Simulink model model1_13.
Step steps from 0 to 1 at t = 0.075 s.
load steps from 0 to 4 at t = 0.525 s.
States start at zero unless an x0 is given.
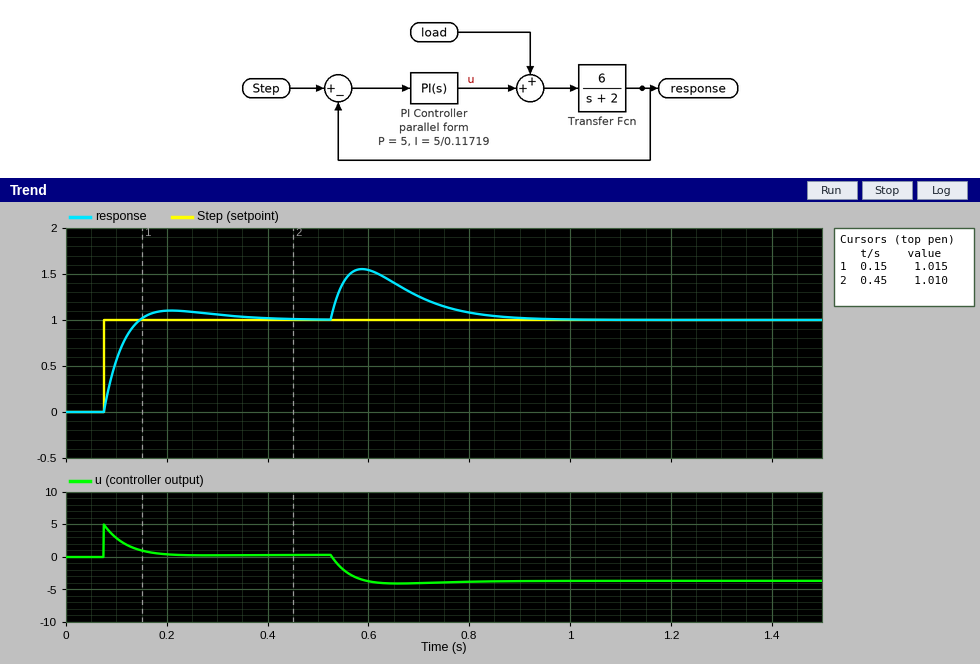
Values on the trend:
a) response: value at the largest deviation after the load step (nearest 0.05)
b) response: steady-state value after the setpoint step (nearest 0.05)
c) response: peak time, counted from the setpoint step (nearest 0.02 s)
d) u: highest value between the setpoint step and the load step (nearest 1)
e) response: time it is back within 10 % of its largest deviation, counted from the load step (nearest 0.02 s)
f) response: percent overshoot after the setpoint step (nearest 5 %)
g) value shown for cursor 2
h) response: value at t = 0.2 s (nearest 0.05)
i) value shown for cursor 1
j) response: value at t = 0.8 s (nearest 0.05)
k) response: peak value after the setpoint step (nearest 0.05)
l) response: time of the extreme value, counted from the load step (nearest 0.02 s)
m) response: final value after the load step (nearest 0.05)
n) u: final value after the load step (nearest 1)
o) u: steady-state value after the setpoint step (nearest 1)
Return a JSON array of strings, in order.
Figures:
["1.55", "1.00", "0.14 s", "5", "0.30 s", "10 %", "1.010", "1.10", "1.015", "1.10", "1.10", "0.06 s", "1.00", "-4", "0"]
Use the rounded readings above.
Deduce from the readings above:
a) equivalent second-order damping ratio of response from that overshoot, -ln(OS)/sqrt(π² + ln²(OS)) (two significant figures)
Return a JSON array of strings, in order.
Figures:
["0.59"]
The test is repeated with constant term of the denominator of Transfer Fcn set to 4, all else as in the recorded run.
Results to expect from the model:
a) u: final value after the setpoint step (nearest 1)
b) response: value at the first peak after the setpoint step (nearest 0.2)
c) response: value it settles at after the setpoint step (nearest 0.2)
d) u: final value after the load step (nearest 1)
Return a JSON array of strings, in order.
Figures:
["1", "1.0", "1.0", "-3"]
